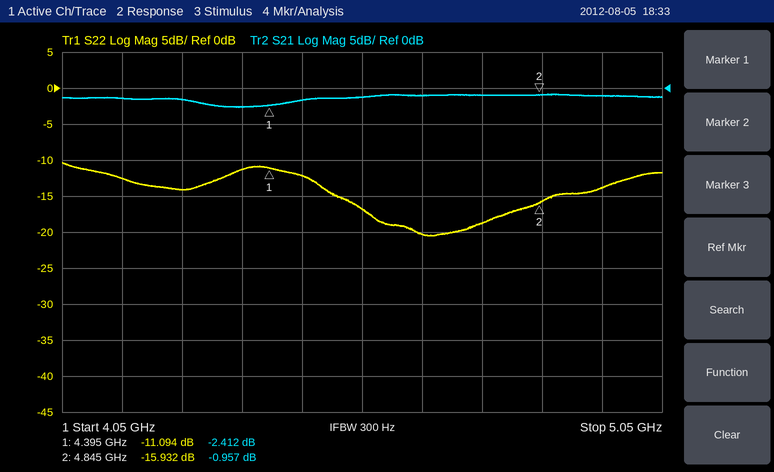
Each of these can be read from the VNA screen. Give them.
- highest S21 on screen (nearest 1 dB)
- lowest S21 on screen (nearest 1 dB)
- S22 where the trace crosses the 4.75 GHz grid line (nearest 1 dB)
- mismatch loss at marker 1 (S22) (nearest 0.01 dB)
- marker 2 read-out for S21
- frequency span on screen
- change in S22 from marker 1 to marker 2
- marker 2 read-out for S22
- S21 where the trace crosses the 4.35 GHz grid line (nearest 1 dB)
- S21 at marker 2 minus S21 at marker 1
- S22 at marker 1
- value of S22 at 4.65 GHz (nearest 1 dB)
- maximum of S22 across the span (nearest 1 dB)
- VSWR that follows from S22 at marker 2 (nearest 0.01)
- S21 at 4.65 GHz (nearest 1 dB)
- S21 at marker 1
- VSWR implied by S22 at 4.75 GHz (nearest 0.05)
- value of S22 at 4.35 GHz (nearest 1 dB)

-1 dB
-3 dB
-19 dB
0.35 dB
-0.957 dB
1 GHz
-4.838 dB
-15.932 dB
-3 dB
1.455 dB
-11.094 dB
-20 dB
-10 dB
1.38
-1 dB
-2.412 dB
1.25
-11 dB
